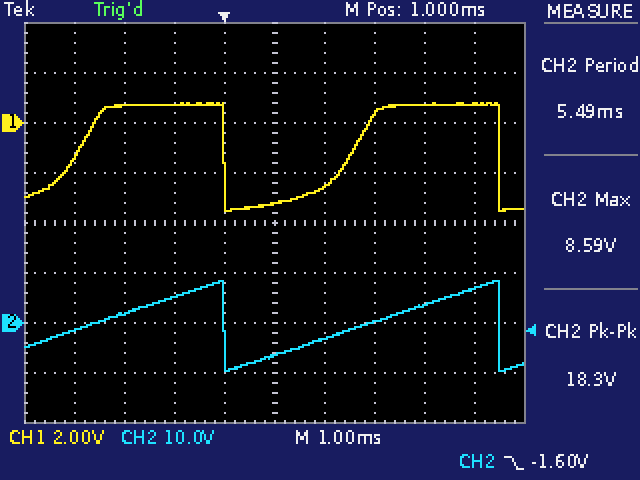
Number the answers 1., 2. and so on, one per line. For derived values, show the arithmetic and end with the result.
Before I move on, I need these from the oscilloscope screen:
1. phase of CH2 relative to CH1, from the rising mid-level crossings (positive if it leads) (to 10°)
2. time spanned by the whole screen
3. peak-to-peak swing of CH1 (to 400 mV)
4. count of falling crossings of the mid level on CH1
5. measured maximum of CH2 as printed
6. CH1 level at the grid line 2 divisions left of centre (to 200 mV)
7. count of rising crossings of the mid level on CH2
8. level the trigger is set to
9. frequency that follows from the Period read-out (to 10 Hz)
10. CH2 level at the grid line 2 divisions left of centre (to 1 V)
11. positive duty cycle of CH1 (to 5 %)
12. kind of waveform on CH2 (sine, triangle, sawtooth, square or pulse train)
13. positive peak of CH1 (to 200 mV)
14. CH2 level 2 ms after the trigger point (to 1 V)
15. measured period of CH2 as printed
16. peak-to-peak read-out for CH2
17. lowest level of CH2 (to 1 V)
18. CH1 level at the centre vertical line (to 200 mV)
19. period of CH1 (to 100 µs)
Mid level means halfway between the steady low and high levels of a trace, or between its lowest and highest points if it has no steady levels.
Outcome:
1. -20°
2. 10 ms
3. 4.4 V
4. 2
5. 8.59 V
6. 800 mV
7. 2
8. -1.60 V
9. 1 / 5.49 ms ≈ 182 Hz, so 180 Hz to the nearest 10 Hz
10. 5 V
11. 55 %
12. sawtooth
13. 800 mV
14. -3 V
15. 5.49 ms
16. 18.3 V
17. -10 V
18. -3.2 V
19. 5.5 ms
